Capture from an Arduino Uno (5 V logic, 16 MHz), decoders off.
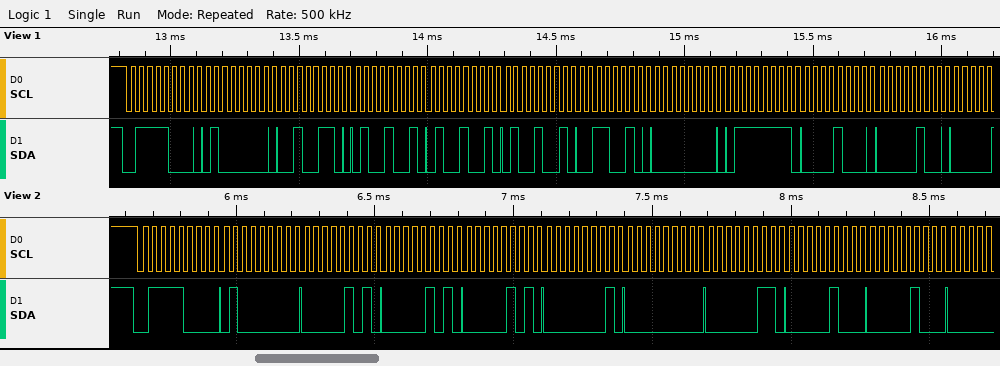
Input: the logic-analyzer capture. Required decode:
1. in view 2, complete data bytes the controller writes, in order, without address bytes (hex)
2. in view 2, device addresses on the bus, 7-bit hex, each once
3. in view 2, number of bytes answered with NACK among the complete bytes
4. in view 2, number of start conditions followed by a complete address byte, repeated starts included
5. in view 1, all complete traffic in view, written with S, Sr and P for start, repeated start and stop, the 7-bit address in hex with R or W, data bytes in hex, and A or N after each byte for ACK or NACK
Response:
40 05 05 05 01 00 03 04 04
0x3C
0
1
S 3CW A 40 A 26 A 49 A 49 A 49 A 32 A 00 A 7F A 08 A 04 A
